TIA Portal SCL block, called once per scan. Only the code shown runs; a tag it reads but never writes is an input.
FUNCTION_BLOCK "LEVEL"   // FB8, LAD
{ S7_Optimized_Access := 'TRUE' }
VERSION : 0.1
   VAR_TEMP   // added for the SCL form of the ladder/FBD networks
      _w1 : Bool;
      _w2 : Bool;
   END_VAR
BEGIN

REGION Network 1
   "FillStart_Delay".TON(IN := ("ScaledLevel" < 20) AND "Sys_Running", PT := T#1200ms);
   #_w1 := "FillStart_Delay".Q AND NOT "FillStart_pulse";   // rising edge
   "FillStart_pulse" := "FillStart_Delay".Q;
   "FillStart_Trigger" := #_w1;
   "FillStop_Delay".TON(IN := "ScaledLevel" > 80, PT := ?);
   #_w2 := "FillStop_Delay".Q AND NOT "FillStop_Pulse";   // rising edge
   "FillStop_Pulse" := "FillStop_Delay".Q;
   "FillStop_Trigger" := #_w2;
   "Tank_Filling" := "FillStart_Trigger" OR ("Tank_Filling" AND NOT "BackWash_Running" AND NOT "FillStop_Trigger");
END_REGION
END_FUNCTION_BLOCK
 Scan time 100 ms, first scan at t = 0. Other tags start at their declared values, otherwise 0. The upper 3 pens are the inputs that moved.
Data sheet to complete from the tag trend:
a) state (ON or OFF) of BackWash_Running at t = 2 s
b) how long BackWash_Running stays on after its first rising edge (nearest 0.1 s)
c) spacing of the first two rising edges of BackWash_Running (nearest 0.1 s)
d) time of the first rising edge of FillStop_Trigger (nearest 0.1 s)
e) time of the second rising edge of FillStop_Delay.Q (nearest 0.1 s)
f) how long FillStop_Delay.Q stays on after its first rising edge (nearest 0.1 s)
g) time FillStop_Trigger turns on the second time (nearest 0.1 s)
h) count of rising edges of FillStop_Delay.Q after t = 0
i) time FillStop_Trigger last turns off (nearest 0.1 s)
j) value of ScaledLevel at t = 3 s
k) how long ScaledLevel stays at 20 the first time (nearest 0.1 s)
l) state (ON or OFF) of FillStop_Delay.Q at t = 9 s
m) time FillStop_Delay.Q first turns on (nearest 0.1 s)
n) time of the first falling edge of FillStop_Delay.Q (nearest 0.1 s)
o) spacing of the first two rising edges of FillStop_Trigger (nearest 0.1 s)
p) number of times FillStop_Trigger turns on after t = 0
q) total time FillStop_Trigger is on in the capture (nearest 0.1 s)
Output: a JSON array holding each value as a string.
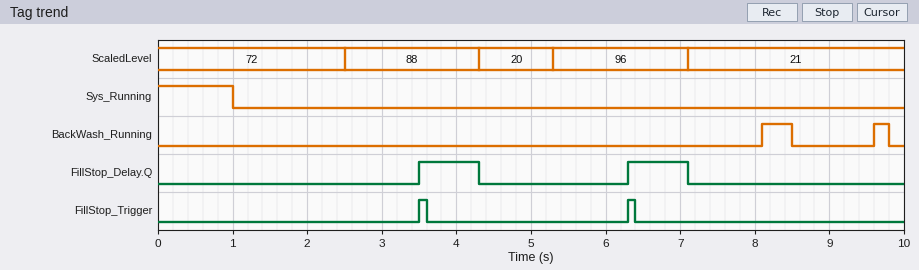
["OFF", "0.4 s", "1.5 s", "3.5 s", "6.3 s", "0.8 s", "6.3 s", "2", "6.4 s", "88", "1.0 s", "OFF", "3.5 s", "4.3 s", "2.8 s", "2", "0.2 s"]
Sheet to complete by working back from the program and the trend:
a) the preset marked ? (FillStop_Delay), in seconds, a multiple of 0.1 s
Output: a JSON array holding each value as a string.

["1.0 s"]
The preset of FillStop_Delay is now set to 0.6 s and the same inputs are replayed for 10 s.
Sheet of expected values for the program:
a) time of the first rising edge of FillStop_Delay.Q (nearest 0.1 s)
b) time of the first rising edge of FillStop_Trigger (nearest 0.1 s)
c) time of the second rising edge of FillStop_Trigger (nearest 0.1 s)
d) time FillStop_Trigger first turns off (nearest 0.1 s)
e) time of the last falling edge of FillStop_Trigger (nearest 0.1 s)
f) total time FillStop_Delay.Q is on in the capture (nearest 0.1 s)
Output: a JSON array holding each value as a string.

["3.1 s", "3.1 s", "5.9 s", "3.2 s", "6.0 s", "2.4 s"]
